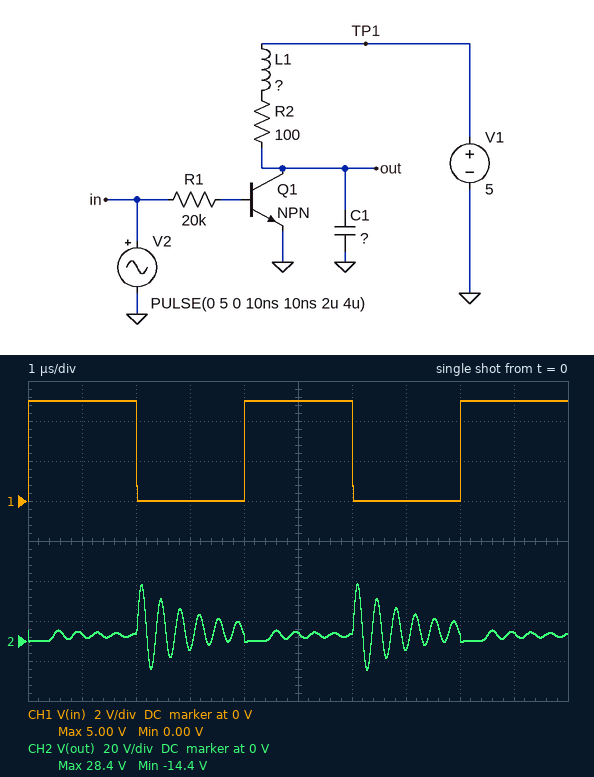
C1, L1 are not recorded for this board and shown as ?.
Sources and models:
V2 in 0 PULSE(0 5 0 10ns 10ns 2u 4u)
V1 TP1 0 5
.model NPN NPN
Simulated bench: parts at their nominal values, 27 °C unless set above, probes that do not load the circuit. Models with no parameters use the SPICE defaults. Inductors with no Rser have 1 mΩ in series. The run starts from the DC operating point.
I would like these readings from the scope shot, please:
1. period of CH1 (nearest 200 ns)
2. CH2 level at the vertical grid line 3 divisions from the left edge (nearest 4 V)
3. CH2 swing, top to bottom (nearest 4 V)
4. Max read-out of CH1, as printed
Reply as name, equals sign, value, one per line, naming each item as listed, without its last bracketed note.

period of CH1 = 4.0 µs
CH2 level at the vertical grid line 3 divisions from the left edge = -4 V
CH2 swing, top to bottom = 44 V
Max read-out of CH1, as printed = 5.00 V
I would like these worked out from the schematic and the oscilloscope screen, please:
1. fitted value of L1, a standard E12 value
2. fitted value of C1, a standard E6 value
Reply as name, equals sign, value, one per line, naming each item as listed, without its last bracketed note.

fitted value of L1, a standard E12 value = 68 µH
fitted value of C1, a standard E6 value = 47 pF
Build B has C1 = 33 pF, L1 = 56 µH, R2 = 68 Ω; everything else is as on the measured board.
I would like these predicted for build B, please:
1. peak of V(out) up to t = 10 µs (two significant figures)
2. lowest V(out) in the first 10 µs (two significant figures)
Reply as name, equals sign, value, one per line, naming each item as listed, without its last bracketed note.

peak of V(out) up to t = 10 µs = 32 V
lowest V(out) in the first 10 µs = -18 V
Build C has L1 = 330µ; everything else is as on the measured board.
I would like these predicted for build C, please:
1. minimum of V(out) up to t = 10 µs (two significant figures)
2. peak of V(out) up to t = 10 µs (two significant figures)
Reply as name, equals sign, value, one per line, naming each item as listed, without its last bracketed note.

minimum of V(out) up to t = 10 µs = -40 V
peak of V(out) up to t = 10 µs = 61 V
